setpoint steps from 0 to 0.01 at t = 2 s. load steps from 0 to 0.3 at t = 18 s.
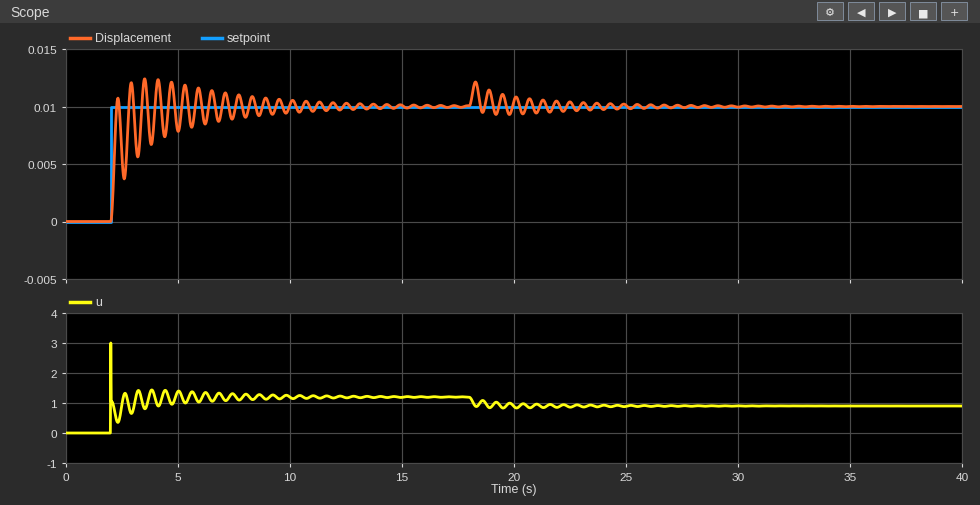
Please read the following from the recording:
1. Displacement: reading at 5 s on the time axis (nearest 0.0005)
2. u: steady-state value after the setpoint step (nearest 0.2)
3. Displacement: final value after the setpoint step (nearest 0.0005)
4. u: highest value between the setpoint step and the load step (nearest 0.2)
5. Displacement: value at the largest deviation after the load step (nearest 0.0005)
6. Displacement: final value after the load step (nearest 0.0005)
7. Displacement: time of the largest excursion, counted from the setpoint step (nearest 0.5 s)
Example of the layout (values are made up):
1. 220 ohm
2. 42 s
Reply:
1. 0.0080
2. 1.2
3. 0.0100
4. 3.0
5. 0.0120
6. 0.0100
7. 1.5 s
